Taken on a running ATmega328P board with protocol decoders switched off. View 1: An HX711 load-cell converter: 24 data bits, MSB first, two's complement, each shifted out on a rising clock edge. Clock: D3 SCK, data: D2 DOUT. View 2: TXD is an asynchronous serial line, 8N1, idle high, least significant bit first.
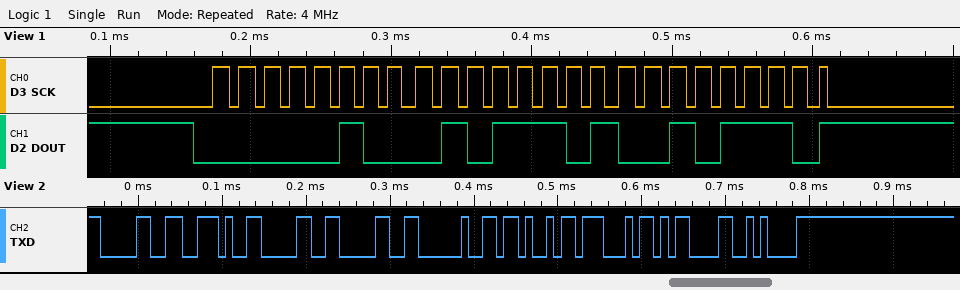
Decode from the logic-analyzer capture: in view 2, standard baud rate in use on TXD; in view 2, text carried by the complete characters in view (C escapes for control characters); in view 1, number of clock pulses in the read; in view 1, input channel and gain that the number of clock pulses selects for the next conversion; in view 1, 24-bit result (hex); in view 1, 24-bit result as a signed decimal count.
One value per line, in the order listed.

115200 baud
"0.00 KG\r\n"
25
channel A, gain 128
0x045D2E
285998
